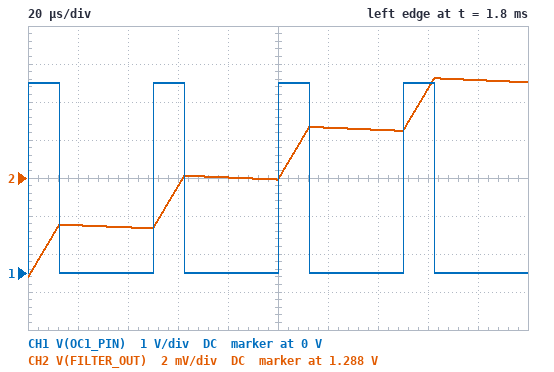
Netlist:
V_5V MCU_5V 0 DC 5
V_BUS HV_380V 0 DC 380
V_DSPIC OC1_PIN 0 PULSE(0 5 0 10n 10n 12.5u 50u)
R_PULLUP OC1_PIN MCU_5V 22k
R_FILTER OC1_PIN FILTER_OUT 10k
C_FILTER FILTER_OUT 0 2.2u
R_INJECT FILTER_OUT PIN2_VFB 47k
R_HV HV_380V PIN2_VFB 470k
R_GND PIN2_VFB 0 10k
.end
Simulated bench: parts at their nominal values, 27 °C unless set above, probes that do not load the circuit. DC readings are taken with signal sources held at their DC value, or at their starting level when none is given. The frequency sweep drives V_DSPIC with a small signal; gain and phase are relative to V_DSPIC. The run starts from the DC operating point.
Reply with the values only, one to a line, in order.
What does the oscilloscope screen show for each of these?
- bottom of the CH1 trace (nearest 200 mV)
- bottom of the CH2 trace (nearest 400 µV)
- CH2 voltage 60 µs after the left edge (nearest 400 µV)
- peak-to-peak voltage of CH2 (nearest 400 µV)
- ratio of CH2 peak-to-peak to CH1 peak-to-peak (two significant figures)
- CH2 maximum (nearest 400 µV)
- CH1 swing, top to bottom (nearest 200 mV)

0 V
1.2828 V
1.2876 V
10.4 mV
0.0021
1.2932 V
5.0 V
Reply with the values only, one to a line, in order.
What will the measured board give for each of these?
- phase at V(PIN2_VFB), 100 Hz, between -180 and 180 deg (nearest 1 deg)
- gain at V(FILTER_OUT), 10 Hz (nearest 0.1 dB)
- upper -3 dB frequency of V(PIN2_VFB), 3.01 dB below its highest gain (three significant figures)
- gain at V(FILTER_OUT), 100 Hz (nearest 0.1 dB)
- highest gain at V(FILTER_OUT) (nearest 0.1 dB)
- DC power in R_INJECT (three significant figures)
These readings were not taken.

-85 deg
-5.2 dB
8.51 Hz
-22.8 dB
-1.4 dB
660 µW
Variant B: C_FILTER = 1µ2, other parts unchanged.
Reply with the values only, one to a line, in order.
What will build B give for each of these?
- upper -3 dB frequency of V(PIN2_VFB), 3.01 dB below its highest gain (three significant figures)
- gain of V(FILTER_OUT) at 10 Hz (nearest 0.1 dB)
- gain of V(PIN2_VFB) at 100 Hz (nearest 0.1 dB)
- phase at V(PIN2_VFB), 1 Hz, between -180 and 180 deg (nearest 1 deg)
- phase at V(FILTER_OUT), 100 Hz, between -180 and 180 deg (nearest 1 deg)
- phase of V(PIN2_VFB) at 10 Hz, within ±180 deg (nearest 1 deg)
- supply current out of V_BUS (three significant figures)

15.6 Hz
-2.9 dB
-32.9 dB
-4 deg
-81 deg
-33 deg
794 µA
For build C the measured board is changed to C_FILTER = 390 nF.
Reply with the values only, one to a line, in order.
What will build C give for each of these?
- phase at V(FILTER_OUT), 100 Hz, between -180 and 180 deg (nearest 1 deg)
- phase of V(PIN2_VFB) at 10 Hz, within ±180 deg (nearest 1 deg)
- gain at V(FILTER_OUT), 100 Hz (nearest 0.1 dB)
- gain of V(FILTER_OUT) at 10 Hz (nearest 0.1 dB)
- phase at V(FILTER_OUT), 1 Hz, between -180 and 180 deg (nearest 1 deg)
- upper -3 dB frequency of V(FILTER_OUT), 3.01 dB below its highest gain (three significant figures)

-64 deg
-12 deg
-8.7 dB
-1.6 dB
-1 deg
48.0 Hz
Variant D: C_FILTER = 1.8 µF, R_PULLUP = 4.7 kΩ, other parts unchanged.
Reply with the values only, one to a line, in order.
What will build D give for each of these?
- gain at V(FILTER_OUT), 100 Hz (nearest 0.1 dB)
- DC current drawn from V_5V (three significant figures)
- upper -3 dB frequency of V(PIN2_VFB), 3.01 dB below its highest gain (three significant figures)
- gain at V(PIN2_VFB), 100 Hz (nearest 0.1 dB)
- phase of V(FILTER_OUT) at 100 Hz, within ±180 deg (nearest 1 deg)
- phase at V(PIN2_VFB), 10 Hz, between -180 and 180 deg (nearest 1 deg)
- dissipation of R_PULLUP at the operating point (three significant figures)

-21.1 dB
1.06 mA
10.4 Hz
-36.4 dB
-84 deg
-44 deg
5.32 mW
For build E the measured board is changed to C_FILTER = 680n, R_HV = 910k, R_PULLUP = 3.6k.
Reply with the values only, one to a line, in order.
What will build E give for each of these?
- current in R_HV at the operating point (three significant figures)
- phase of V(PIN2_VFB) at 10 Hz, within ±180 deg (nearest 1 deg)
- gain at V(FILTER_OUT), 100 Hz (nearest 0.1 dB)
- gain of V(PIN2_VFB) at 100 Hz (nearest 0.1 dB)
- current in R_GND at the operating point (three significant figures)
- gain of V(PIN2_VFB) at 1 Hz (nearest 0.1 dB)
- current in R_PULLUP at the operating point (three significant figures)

414 µA
-20 deg
-12.9 dB
-28.1 dB
352 µA
-16.6 dB
1.39 mA
